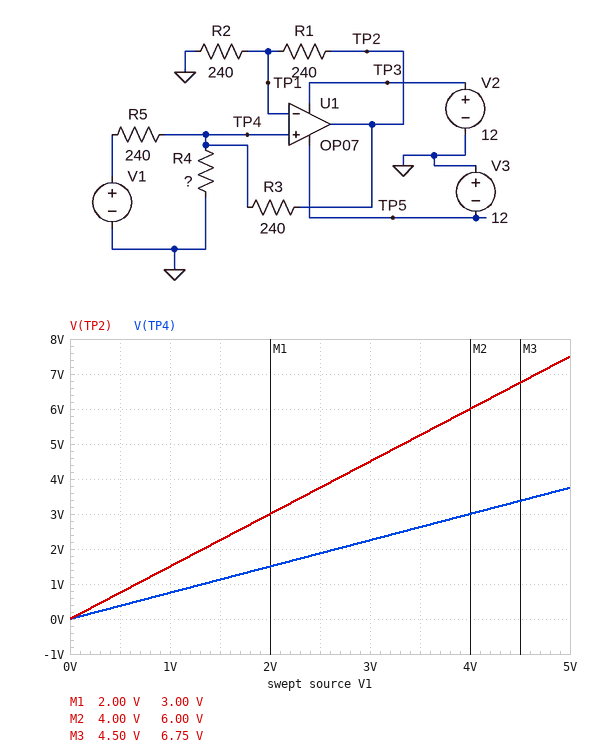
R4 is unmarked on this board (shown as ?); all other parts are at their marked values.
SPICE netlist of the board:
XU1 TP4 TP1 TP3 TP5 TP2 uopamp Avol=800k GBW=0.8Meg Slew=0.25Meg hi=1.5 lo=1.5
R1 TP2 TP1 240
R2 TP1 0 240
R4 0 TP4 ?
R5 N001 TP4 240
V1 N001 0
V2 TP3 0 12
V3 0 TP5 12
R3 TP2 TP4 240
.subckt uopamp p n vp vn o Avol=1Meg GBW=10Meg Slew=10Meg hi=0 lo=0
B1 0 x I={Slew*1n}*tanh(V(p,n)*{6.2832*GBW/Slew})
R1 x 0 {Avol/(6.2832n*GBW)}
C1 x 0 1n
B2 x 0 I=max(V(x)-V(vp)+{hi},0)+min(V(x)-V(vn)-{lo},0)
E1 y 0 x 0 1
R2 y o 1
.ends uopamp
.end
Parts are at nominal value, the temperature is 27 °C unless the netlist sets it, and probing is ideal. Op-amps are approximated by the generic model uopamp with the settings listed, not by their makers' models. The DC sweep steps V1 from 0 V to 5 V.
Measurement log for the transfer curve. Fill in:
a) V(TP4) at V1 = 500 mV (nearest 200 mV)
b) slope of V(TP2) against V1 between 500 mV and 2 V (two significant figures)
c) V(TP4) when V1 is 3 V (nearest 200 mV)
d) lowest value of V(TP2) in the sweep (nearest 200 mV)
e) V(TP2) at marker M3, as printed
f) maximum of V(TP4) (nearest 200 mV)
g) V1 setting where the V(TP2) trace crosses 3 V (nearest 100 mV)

400 mV
1.5 V/V
2.2 V
0 V
6.75 V
3.8 V
2.0 V
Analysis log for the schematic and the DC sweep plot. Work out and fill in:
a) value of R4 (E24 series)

180 Ω
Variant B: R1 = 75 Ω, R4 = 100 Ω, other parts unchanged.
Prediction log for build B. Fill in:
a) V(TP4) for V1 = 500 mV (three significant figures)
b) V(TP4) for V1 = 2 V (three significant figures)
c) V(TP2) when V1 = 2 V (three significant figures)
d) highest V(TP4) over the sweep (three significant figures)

162 mV
648 mV
850 mV
1.62 V
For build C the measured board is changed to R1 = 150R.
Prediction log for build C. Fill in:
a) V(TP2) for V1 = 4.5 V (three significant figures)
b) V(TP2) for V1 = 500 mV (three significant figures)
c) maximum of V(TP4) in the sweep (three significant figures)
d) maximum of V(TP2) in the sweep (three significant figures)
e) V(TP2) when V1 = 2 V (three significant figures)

4.28 V
476 mV
2.93 V
4.76 V
1.90 V
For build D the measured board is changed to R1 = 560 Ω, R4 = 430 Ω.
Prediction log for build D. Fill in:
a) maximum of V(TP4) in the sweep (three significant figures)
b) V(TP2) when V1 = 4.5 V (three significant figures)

6.05 V
10.5 V
